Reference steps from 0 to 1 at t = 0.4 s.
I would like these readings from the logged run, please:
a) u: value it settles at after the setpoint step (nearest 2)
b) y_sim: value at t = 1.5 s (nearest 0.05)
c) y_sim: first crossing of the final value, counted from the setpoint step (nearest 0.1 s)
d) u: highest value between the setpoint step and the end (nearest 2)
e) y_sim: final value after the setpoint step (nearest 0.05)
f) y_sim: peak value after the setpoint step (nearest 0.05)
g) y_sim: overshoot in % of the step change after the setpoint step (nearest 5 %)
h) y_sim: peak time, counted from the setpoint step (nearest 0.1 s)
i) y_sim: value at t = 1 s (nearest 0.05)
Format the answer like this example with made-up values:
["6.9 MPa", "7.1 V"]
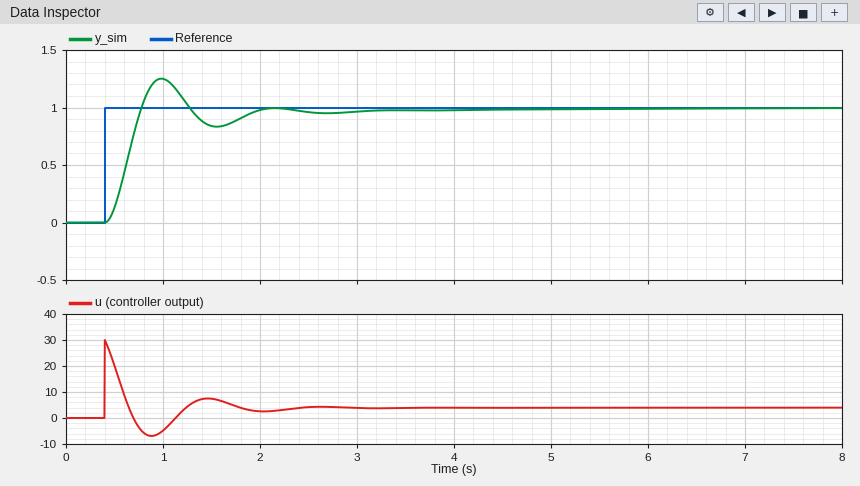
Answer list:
["4", "0.85", "0.4 s", "30", "1.00", "1.25", "25 %", "0.6 s", "1.25"]
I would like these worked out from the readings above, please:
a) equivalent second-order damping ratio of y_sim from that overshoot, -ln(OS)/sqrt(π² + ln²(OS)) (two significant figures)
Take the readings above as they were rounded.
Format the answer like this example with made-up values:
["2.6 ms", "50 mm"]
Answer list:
["0.40"]
